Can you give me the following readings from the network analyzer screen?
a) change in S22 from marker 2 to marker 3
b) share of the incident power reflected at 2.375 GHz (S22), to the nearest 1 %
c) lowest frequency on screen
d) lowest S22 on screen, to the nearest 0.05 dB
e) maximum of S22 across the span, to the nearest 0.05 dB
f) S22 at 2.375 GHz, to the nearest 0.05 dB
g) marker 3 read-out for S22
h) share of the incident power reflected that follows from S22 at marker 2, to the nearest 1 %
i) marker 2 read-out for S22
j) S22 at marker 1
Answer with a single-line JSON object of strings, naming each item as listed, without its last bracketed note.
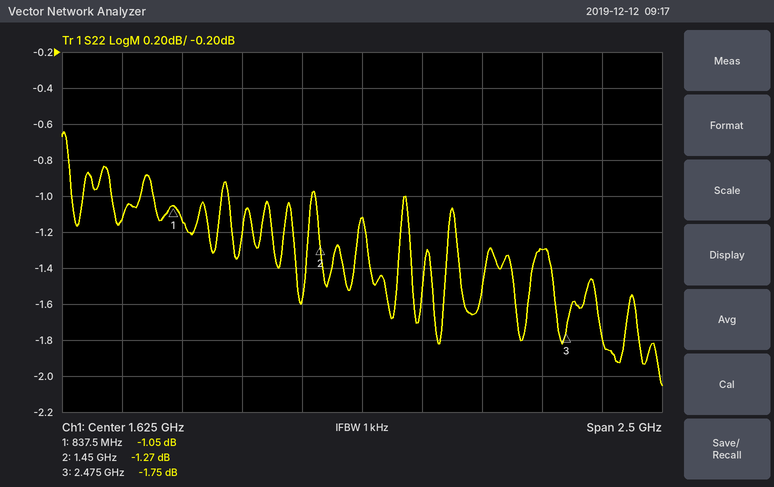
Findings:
{"change in S22 from marker 2 to marker 3": "-0.48 dB", "share of the incident power reflected at 2.375 GHz (S22), to the nearest 1 %": "74 %", "lowest frequency on screen": "375 MHz", "lowest S22 on screen, to the nearest 0.05 dB": "-2.05 dB", "maximum of S22 across the span, to the nearest 0.05 dB": "-0.65 dB", "S22 at 2.375 GHz, to the nearest 0.05 dB": "-1.30 dB", "marker 3 read-out for S22": "-1.75 dB", "share of the incident power reflected that follows from S22 at marker 2, to the nearest 1 %": "75 %", "marker 2 read-out for S22": "-1.27 dB", "S22 at marker 1": "-1.05 dB"}
